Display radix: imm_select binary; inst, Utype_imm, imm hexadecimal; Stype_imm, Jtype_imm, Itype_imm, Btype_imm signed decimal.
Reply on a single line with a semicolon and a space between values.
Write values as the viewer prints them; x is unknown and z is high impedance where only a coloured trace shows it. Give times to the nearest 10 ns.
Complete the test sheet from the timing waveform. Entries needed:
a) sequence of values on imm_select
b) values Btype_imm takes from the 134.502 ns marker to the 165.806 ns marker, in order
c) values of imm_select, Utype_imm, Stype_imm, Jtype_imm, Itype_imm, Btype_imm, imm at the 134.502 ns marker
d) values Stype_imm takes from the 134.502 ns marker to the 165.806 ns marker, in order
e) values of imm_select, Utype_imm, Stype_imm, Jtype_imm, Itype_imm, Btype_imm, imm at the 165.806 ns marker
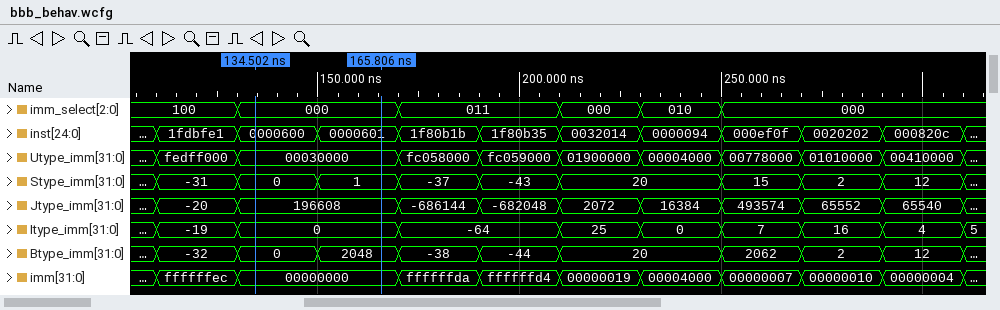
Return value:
100, 000, 011, 000, 010, 000; 0, 2048; imm_select=000, Utype_imm=00030000, Stype_imm=0, Jtype_imm=196608, Itype_imm=0, Btype_imm=0, imm=00000000; 0, 1; imm_select=000, Utype_imm=00030000, Stype_imm=1, Jtype_imm=196608, Itype_imm=0, Btype_imm=2048, imm=00000000
